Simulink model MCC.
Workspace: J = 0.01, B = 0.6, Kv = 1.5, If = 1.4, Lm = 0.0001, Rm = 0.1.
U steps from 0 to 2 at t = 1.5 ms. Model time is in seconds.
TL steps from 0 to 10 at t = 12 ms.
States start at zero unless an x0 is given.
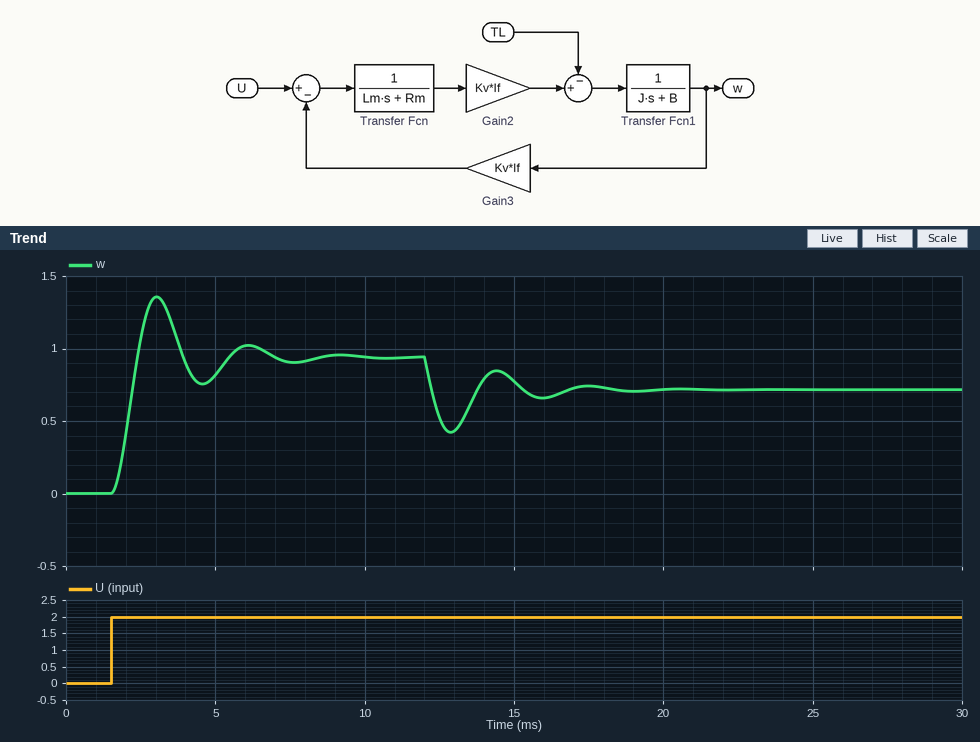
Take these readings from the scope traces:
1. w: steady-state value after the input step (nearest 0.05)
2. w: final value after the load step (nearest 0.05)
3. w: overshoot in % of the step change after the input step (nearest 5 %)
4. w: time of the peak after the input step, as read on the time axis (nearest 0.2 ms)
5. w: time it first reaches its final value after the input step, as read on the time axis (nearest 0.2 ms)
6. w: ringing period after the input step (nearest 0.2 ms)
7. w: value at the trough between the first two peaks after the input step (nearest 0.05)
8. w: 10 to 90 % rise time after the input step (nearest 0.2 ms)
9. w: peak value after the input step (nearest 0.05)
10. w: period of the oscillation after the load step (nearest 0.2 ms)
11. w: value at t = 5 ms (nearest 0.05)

0.95
0.70
45 %
3.0 ms
2.4 ms
3.0 ms
0.75
0.6 ms
1.35
3.0 ms
0.80
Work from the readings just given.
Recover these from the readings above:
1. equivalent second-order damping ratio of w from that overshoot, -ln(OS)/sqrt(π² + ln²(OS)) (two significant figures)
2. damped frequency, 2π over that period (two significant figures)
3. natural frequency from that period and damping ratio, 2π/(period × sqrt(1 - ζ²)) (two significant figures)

0.25
2.1 rad/ms
2.2 rad/ms
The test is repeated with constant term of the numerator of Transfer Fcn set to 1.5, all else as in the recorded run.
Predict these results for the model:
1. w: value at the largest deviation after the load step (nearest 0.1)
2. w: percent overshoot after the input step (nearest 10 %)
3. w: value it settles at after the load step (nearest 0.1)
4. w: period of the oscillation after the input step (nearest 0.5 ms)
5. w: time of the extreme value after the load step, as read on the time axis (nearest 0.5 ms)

0.5
50 %
0.8
2.5 ms
12.5 ms
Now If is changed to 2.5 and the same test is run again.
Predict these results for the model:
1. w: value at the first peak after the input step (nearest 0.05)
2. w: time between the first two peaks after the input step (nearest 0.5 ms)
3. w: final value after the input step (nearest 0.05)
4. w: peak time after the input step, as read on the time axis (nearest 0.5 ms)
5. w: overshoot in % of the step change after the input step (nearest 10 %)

0.85
1.5 ms
0.55
2.5 ms
60 %
